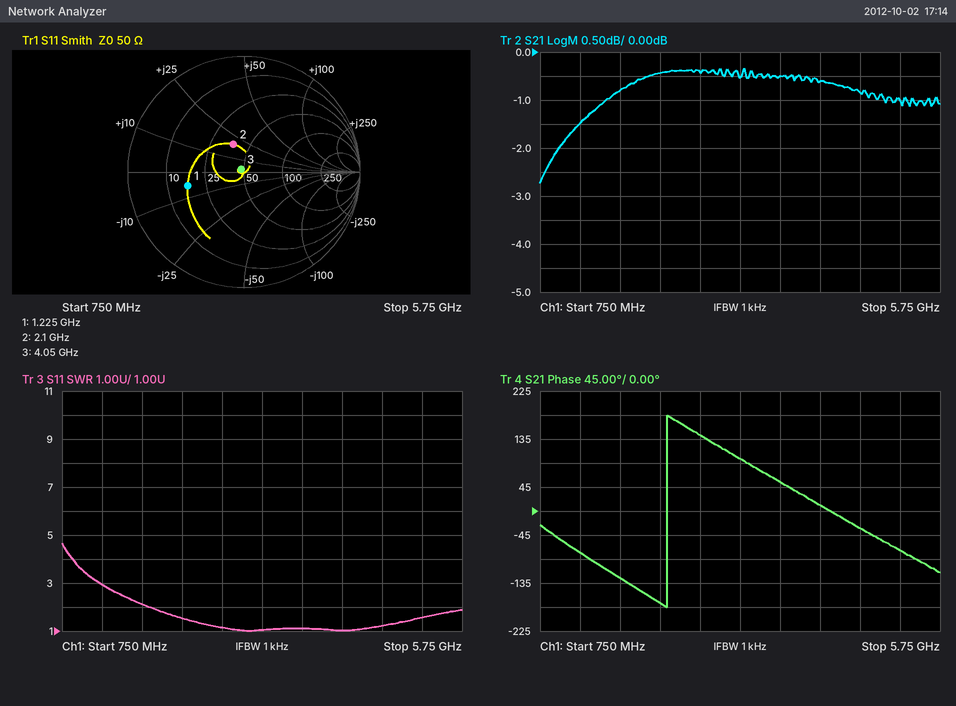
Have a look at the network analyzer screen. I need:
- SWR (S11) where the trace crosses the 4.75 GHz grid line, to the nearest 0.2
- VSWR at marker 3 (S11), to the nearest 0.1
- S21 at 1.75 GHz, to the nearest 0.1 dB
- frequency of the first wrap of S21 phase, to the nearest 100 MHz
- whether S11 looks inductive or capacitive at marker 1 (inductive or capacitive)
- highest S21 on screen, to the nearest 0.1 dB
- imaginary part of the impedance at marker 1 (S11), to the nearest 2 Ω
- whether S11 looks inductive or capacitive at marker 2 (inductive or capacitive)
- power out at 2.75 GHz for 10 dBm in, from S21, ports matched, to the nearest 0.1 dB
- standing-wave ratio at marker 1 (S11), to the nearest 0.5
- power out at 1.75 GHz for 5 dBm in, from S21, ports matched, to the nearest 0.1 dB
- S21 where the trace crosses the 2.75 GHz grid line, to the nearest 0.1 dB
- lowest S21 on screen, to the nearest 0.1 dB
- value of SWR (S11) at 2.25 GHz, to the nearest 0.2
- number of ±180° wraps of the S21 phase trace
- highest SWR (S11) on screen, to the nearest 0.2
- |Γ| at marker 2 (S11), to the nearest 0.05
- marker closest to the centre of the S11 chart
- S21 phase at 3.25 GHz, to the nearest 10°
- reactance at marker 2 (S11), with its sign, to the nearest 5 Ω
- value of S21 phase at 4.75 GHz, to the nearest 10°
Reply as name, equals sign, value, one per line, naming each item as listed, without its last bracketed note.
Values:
SWR (S11) where the trace crosses the 4.75 GHz grid line, to the nearest 0.2 = 1.2
VSWR at marker 3 (S11), to the nearest 0.1 = 1.1
S21 at 1.75 GHz, to the nearest 0.1 dB = -0.8 dB
frequency of the first wrap of S21 phase, to the nearest 100 MHz = 2.3 GHz
whether S11 looks inductive or capacitive at marker 1 = capacitive
highest S21 on screen, to the nearest 0.1 dB = -0.3 dB
imaginary part of the impedance at marker 1 (S11), to the nearest 2 Ω = -6 Ω
whether S11 looks inductive or capacitive at marker 2 = inductive
power out at 2.75 GHz for 10 dBm in, from S21, ports matched, to the nearest 0.1 dB = 9.6 dBm
standing-wave ratio at marker 1 (S11), to the nearest 0.5 = 3.0
power out at 1.75 GHz for 5 dBm in, from S21, ports matched, to the nearest 0.1 dB = 4.2 dBm
S21 where the trace crosses the 2.75 GHz grid line, to the nearest 0.1 dB = -0.4 dB
lowest S21 on screen, to the nearest 0.1 dB = -2.7 dB
value of SWR (S11) at 2.25 GHz, to the nearest 0.2 = 1.6
number of ±180° wraps of the S21 phase trace = 1
highest SWR (S11) on screen, to the nearest 0.2 = 4.6
|Γ| at marker 2 (S11), to the nearest 0.05 = 0.25
marker closest to the centre of the S11 chart = marker 3
S21 phase at 3.25 GHz, to the nearest 10° = 100°
reactance at marker 2 (S11), with its sign, to the nearest 5 Ω = +20 Ω
value of S21 phase at 4.75 GHz, to the nearest 10° = -30°
